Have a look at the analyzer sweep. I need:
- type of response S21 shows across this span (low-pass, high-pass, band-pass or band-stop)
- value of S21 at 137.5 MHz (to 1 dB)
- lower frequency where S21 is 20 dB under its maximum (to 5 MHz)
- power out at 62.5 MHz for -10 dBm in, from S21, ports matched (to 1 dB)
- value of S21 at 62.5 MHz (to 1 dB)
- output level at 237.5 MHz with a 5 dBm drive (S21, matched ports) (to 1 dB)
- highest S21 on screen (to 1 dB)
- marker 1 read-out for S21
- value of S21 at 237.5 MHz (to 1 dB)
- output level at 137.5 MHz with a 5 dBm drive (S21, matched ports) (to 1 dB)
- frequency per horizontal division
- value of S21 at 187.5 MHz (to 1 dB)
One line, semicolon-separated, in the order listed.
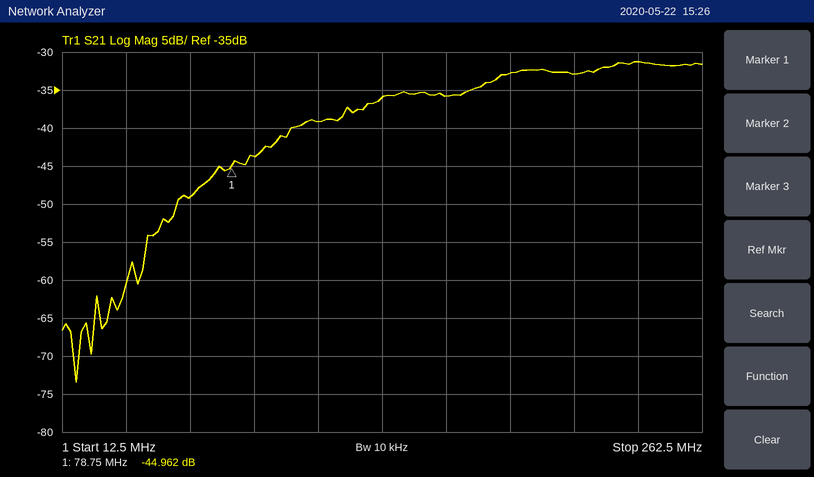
high-pass; -36 dB; 55 MHz; -59 dBm; -49 dB; -26 dBm; -31 dB; -44.962 dB; -31 dB; -31 dBm; 25 MHz; -33 dB
